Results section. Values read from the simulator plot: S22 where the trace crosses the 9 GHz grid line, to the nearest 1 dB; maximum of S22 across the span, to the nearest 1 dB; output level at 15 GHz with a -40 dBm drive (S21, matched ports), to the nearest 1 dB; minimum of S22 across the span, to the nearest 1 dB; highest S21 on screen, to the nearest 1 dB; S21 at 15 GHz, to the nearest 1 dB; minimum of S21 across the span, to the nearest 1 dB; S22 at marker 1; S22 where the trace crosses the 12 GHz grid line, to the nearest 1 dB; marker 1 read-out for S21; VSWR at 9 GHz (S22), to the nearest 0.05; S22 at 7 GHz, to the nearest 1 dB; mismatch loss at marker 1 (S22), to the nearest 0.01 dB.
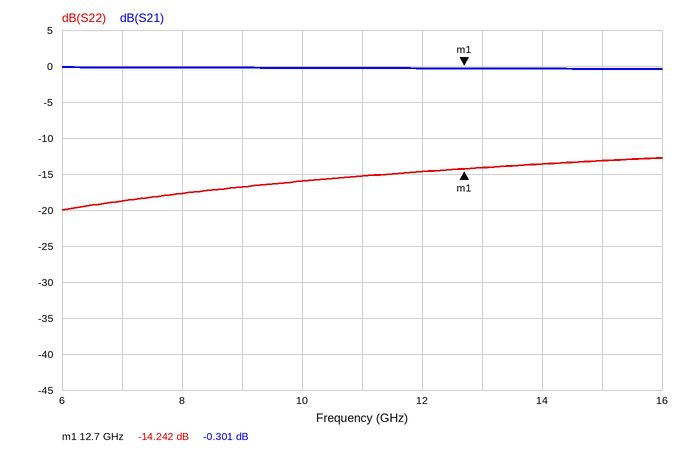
-17 dB
-13 dB
-40 dBm
-20 dB
0 dB
0 dB
0 dB
-14.242 dB
-15 dB
-0.301 dB
1.35
-19 dB
0.17 dB
